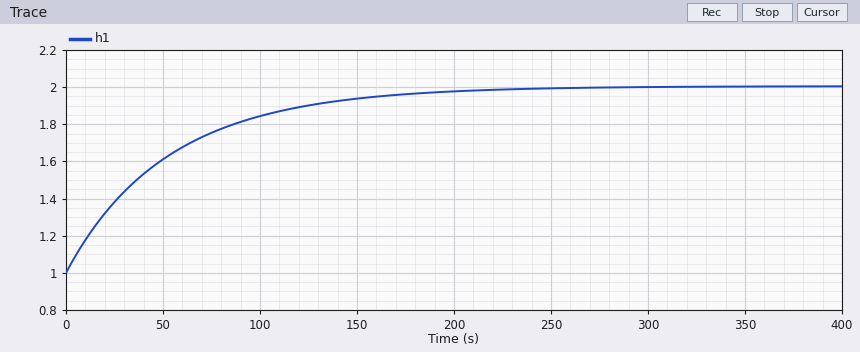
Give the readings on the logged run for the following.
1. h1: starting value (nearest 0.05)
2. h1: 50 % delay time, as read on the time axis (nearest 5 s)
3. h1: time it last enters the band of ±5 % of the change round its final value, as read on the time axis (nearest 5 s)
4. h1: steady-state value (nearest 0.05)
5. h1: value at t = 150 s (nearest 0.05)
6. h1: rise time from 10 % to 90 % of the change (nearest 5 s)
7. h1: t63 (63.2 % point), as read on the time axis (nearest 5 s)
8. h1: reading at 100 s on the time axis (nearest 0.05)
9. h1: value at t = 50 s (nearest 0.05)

1.00
35 s
165 s
2.00
1.95
120 s
55 s
1.85
1.60
